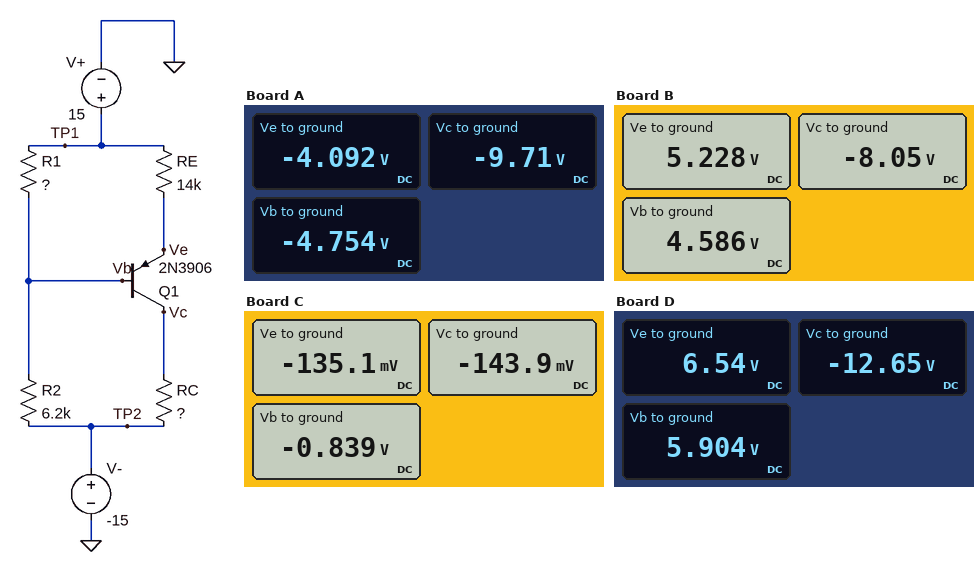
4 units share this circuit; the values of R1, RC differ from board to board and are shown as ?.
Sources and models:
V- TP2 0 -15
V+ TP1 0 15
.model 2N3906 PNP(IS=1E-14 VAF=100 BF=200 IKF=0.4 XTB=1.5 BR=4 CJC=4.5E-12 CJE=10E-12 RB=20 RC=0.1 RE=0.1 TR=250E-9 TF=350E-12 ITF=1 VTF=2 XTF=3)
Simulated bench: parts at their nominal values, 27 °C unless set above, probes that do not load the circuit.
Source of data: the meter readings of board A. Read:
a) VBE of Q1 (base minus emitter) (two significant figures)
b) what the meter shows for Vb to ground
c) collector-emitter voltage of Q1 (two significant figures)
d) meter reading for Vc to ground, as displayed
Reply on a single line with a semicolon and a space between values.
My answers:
-660 mV; -4.754 V; -5.6 V; -9.71 V
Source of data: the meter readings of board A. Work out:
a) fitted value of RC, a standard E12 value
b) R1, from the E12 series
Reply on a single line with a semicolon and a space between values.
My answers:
3.9 kΩ; 12 kΩ
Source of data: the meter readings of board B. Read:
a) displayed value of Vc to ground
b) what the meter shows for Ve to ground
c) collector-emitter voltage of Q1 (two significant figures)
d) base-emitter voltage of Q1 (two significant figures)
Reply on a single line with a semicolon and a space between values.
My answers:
-8.05 V; 5.228 V; -13 V; -640 mV
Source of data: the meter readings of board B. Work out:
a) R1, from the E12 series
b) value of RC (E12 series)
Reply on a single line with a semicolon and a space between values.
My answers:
3.3 kΩ; 10 kΩ
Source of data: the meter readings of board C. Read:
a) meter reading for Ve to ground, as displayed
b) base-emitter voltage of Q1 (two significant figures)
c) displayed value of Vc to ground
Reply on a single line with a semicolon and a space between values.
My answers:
-135.1 mV; -700 mV; -143.9 mV
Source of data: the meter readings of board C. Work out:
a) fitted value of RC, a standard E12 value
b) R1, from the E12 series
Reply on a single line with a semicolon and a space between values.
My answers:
39 kΩ; 10 kΩ
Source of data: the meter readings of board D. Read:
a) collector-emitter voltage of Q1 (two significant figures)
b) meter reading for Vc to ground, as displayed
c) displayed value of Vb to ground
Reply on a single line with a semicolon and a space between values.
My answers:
-19 V; -12.65 V; 5.904 V
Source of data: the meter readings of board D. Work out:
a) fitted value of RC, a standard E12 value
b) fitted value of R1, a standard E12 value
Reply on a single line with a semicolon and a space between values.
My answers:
3.9 kΩ; 2.7 kΩ
